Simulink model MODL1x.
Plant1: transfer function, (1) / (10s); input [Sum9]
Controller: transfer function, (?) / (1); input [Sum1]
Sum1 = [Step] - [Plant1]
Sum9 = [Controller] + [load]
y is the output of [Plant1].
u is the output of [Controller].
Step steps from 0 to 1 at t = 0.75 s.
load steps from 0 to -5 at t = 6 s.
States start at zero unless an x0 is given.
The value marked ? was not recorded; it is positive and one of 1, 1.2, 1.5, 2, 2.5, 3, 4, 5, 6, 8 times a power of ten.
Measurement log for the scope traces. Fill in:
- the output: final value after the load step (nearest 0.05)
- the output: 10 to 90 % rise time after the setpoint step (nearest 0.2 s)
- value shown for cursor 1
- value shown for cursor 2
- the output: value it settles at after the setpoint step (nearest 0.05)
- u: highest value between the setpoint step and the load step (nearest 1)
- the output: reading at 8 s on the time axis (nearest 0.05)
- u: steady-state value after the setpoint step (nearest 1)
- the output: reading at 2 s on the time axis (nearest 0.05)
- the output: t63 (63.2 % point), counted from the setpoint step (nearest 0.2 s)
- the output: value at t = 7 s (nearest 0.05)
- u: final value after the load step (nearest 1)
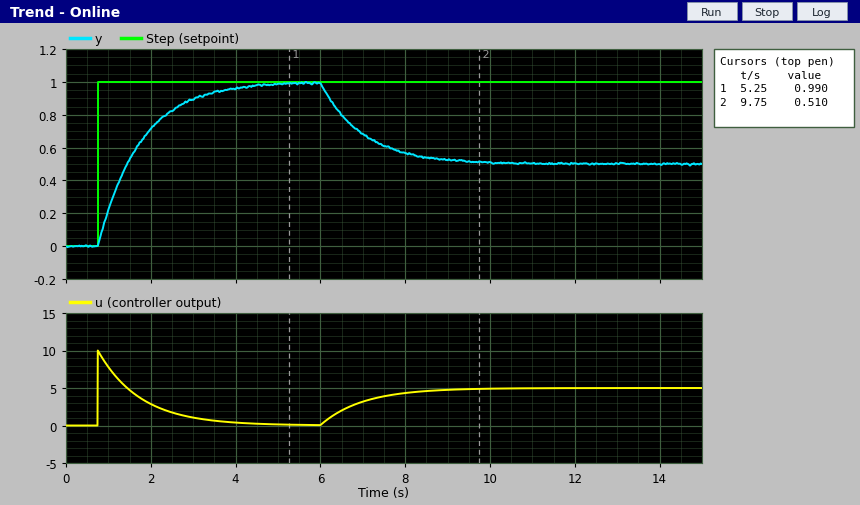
0.50
2.2 s
0.990
0.510
1.00
10
0.55
0
0.70
1.0 s
0.70
5
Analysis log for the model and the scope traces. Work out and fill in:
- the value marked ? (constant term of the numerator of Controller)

10
